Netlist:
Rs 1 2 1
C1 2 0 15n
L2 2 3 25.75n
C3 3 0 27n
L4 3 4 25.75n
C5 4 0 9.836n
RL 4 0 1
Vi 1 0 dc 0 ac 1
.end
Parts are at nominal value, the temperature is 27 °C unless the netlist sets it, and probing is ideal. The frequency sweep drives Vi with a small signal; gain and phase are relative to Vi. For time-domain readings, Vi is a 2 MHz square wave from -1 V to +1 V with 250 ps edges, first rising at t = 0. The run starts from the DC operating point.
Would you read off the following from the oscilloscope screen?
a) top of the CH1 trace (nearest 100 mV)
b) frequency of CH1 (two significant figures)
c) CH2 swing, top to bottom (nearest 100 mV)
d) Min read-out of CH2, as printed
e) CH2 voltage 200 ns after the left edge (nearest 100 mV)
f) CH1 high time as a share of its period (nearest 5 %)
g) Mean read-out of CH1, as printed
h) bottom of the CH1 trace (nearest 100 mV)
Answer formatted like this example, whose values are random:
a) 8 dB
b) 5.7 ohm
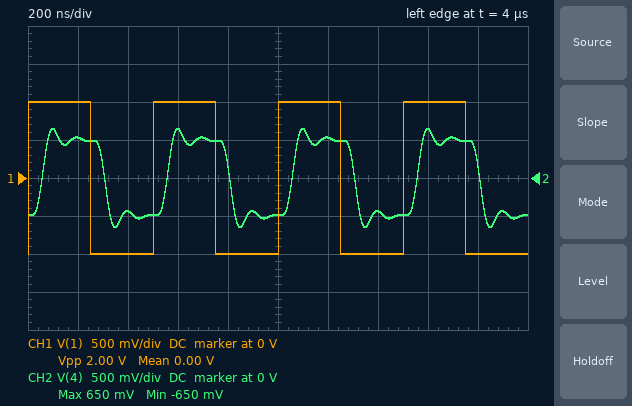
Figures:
a) 1.0 V
b) 2.0 MHz
c) 1.3 V
d) -650 mV
e) 500 mV
f) 50 %
g) 0.00 V
h) -1.0 V
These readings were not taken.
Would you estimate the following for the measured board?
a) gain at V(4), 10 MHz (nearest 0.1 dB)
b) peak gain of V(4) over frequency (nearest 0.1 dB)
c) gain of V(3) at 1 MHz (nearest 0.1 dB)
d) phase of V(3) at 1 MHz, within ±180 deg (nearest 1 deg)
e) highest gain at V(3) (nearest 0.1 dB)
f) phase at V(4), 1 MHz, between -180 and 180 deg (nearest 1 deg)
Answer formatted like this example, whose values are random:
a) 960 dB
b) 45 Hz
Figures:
a) -6.9 dB
b) -6.0 dB
c) -6.0 dB
d) -9 deg
e) -2.6 dB
f) -19 deg
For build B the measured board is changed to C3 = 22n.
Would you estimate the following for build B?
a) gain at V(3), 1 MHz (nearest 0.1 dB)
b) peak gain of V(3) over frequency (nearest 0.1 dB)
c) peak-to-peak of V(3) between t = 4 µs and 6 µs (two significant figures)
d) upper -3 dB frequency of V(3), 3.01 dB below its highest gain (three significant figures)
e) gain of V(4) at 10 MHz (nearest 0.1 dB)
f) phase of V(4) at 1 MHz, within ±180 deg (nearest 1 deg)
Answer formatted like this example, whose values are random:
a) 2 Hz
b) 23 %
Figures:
a) -6.0 dB
b) -1.6 dB
c) 1.6 V
d) 12.5 MHz
e) -6.0 dB
f) -18 deg
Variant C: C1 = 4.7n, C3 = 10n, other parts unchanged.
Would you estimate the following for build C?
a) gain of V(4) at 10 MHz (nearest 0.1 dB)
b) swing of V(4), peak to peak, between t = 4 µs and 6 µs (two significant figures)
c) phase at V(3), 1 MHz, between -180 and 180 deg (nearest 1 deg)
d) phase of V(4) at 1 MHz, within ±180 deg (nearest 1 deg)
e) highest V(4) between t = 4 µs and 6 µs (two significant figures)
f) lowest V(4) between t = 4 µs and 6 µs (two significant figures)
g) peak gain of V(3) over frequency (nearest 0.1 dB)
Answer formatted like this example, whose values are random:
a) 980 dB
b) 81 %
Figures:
a) -7.7 dB
b) 1.1 V
c) -4 deg
d) -14 deg
e) 560 mV
f) -560 mV
g) 2.6 dB
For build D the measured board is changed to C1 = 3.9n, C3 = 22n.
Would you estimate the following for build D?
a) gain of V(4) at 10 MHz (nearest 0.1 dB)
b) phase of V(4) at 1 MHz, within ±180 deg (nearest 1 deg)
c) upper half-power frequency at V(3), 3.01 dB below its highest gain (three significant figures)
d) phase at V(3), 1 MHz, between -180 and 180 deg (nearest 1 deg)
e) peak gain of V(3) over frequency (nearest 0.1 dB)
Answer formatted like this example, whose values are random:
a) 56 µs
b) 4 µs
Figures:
a) -6.6 dB
b) -16 deg
c) 12.8 MHz
d) -6 deg
e) -2.4 dB
